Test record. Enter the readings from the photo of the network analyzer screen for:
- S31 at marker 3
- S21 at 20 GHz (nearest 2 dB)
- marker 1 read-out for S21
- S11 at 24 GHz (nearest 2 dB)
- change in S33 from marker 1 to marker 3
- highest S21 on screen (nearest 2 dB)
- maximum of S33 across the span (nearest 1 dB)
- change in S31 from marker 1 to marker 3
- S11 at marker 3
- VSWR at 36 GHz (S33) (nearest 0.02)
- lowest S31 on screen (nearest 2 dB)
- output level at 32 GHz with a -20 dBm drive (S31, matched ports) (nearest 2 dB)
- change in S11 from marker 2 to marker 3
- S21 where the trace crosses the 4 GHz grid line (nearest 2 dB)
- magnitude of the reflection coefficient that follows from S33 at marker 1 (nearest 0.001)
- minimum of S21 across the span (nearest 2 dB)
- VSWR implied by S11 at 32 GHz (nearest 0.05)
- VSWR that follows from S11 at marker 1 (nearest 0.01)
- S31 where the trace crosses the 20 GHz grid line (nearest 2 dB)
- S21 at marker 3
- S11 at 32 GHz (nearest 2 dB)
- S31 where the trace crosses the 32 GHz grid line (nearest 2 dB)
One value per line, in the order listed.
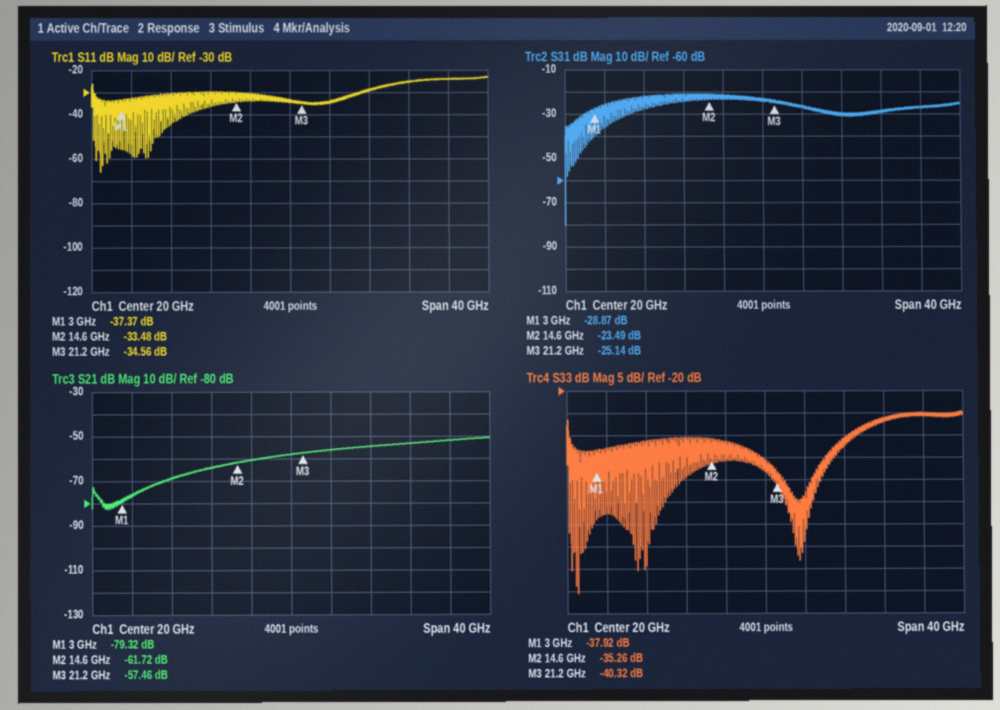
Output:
-25.14 dB
-58 dB
-79.32 dB
-34 dB
-2.40 dB
-50 dB
-25 dB
3.73 dB
-34.56 dB
1.12
-80 dB
-48 dBm
-1.08 dB
-76 dB
0.013
-82 dB
1.10
1.03
-24 dB
-57.46 dB
-26 dB
-28 dB
